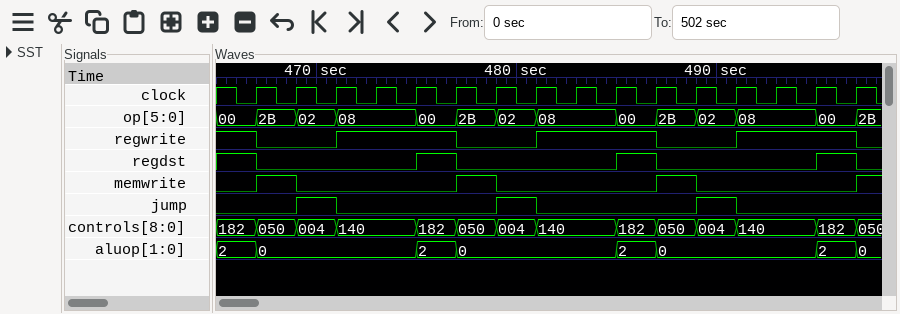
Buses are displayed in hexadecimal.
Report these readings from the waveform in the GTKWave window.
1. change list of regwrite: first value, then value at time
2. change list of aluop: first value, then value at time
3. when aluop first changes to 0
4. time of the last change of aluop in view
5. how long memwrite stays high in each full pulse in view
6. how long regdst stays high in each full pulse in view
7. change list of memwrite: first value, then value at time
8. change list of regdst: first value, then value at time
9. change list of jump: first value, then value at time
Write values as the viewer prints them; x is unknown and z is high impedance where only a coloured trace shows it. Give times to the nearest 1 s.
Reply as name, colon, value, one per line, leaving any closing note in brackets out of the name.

change list of regwrite: first value, then value at time: 1, 0 at 467 s, 1 at 471 s, 0 at 477 s, 1 at 481 s, 0 at 487 s, 1 at 491 s, 0 at 497 s
change list of aluop: first value, then value at time: 2, 0 at 467 s, 2 at 475 s, 0 at 477 s, 2 at 485 s, 0 at 487 s, 2 at 495 s, 0 at 497 s
when aluop first changes to 0: 467 s
time of the last change of aluop in view: 497 s
how long memwrite stays high in each full pulse in view: 2 s, 2 s, 2 s
how long regdst stays high in each full pulse in view: 2 s, 2 s, 2 s
change list of memwrite: first value, then value at time: 0, 1 at 467 s, 0 at 469 s, 1 at 477 s, 0 at 479 s, 1 at 487 s, 0 at 489 s, 1 at 497 s
change list of regdst: first value, then value at time: 1, 0 at 467 s, 1 at 475 s, 0 at 477 s, 1 at 485 s, 0 at 487 s, 1 at 495 s, 0 at 497 s
change list of jump: first value, then value at time: 0, 1 at 469 s, 0 at 471 s, 1 at 479 s, 0 at 481 s, 1 at 489 s, 0 at 491 s
